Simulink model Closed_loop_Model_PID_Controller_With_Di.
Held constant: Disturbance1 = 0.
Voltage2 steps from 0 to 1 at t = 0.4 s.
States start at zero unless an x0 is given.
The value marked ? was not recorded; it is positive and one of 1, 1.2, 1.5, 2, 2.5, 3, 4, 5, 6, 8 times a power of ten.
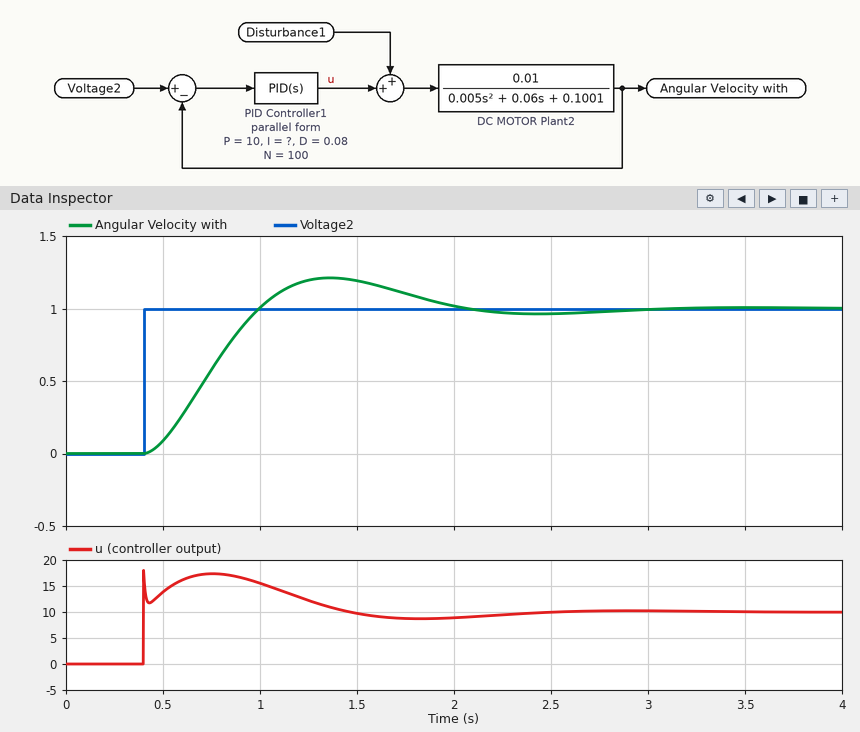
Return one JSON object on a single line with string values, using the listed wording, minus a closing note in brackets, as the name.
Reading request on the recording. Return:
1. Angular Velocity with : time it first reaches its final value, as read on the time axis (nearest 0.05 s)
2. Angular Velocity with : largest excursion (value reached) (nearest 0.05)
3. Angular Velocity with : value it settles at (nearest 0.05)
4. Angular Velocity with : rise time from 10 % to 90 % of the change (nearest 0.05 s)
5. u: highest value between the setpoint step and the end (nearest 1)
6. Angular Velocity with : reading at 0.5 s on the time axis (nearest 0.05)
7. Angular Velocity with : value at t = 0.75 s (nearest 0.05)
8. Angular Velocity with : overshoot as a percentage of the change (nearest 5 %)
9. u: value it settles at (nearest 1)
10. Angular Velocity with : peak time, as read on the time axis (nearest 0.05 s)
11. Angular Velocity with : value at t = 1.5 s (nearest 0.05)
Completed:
{"Angular Velocity with : time it first reaches its final value, as read on the time axis": "1.00 s", "Angular Velocity with : largest excursion (value reached)": "1.20", "Angular Velocity with : value it settles at": "1.00", "Angular Velocity with : rise time from 10 % to 90 % of the change": "0.40 s", "u: highest value between the setpoint step and the end": "18", "Angular Velocity with : reading at 0.5 s on the time axis": "0.10", "Angular Velocity with : value at t = 0.75 s": "0.60", "Angular Velocity with : overshoot as a percentage of the change": "20 %", "u: value it settles at": "10", "Angular Velocity with : peak time, as read on the time axis": "1.35 s", "Angular Velocity with : value at t = 1.5 s": "1.20"}
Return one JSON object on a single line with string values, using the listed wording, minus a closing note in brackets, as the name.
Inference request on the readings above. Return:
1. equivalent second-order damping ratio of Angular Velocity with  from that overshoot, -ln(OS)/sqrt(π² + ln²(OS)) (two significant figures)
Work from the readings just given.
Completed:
{"equivalent second-order damping ratio of Angular Velocity with  from that overshoot, -ln(OS)/sqrt(π² + ln²(OS))": "0.46"}
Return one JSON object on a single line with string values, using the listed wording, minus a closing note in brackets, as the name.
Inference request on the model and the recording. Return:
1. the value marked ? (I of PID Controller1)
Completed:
{"the value marked ?": "50"}
